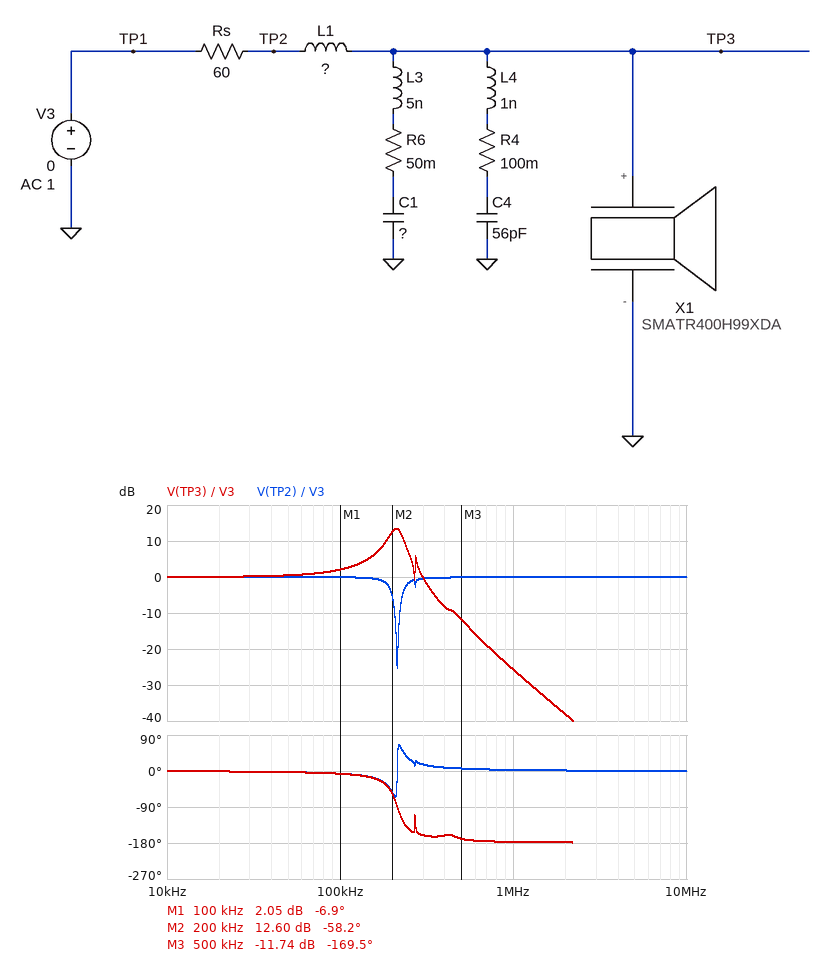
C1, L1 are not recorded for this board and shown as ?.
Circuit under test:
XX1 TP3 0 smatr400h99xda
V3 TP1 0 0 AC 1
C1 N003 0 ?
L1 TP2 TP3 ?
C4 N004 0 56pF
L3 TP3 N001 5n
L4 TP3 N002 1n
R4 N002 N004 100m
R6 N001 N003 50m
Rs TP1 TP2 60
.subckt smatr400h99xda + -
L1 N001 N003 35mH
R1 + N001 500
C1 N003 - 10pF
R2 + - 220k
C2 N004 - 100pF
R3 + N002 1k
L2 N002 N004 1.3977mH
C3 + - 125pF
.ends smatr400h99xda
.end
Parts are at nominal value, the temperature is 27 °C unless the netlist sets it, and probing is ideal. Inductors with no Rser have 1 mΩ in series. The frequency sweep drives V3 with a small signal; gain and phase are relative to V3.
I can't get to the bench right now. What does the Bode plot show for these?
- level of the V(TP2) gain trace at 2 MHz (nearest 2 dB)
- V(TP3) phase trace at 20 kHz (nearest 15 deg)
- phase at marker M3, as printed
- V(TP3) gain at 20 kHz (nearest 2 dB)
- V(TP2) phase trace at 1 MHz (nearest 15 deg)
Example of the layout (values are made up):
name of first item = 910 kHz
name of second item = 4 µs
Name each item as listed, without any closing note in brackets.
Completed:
level of the V(TP2) gain trace at 2 MHz = 0 dB
V(TP3) phase trace at 20 kHz = 0 deg
phase at marker M3, as printed = -169.5 deg
V(TP3) gain at 20 kHz = 0 dB
V(TP2) phase trace at 1 MHz = 0 deg
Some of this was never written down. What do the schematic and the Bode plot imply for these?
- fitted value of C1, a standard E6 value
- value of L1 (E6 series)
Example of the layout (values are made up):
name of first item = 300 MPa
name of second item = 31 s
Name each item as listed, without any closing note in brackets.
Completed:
fitted value of C1, a standard E6 value = 2.2 nF
value of L1 = 220 µH
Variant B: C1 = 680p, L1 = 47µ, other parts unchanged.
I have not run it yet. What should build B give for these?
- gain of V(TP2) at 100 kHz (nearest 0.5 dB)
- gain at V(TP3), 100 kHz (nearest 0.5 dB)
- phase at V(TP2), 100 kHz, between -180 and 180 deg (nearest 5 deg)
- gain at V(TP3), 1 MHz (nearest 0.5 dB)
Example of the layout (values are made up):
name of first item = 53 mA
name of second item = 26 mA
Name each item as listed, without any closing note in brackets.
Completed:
gain of V(TP2) at 100 kHz = 0 dB
gain at V(TP3), 100 kHz = 0 dB
phase at V(TP2), 100 kHz, between -180 and 180 deg = 0 deg
gain at V(TP3), 1 MHz = 4.0 dB
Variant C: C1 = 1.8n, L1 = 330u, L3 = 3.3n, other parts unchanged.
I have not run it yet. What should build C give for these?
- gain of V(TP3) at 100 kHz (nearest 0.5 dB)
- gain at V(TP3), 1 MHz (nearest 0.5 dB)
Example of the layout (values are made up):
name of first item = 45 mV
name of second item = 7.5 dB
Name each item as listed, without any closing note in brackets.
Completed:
gain of V(TP3) at 100 kHz = 2.5 dB
gain at V(TP3), 1 MHz = -28.0 dB
